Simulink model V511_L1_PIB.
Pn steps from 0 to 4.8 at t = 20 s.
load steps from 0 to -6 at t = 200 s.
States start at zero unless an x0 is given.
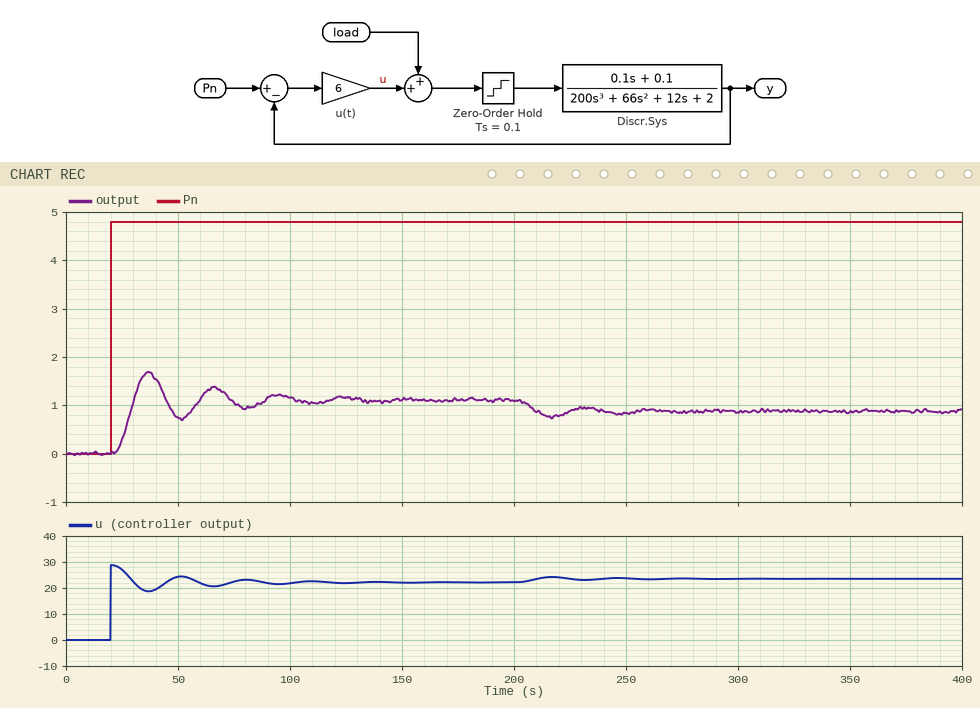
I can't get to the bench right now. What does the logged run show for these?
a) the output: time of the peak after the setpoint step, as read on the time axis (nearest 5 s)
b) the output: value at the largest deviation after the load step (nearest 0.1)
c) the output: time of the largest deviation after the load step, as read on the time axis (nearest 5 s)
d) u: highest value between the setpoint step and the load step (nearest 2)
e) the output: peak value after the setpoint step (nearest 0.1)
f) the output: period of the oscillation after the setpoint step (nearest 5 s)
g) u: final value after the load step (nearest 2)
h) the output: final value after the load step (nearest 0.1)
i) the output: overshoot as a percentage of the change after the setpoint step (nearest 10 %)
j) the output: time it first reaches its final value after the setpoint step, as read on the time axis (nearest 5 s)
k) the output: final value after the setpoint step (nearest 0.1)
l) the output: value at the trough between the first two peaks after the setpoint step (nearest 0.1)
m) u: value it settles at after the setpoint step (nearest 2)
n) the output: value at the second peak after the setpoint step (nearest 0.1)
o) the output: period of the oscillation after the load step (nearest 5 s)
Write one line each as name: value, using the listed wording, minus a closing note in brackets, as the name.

the output: time of the peak after the setpoint step, as read on the time axis: 35 s
the output: value at the largest deviation after the load step: 0.8
the output: time of the largest deviation after the load step, as read on the time axis: 215 s
u: highest value between the setpoint step and the load step: 28
the output: peak value after the setpoint step: 1.7
the output: period of the oscillation after the setpoint step: 30 s
u: final value after the load step: 24
the output: final value after the load step: 0.9
the output: overshoot as a percentage of the change after the setpoint step: 50 %
the output: time it first reaches its final value after the setpoint step, as read on the time axis: 30 s
the output: final value after the setpoint step: 1.1
the output: value at the trough between the first two peaks after the setpoint step: 0.7
u: value it settles at after the setpoint step: 22
the output: value at the second peak after the setpoint step: 1.4
the output: period of the oscillation after the load step: 30 s
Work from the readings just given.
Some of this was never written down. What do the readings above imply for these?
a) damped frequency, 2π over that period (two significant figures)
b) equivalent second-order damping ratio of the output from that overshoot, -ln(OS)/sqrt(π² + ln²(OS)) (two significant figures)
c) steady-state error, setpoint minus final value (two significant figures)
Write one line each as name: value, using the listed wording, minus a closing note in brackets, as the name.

damped frequency, 2π over that period: 0.21 rad/s
equivalent second-order damping ratio of the output from that overshoot, -ln(OS)/sqrt(π² + ln²(OS)): 0.22
steady-state error, setpoint minus final value: 3.7
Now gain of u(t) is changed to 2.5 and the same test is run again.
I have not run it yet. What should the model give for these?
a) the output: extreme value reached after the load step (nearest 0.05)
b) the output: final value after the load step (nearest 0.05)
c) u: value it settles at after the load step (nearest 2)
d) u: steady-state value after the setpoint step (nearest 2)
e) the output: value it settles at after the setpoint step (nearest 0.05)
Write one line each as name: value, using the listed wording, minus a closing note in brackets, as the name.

the output: extreme value reached after the load step: 0.15
the output: final value after the load step: 0.25
u: value it settles at after the load step: 12
u: steady-state value after the setpoint step: 10
the output: value it settles at after the setpoint step: 0.55
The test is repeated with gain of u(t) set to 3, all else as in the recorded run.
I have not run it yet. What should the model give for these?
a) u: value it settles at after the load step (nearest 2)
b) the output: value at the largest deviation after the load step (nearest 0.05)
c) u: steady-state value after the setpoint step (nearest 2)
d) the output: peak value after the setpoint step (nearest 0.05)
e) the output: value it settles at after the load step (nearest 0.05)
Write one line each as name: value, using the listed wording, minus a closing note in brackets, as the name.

u: value it settles at after the load step: 14
the output: value at the largest deviation after the load step: 0.25
u: steady-state value after the setpoint step: 12
the output: peak value after the setpoint step: 0.90
the output: value it settles at after the load step: 0.35
